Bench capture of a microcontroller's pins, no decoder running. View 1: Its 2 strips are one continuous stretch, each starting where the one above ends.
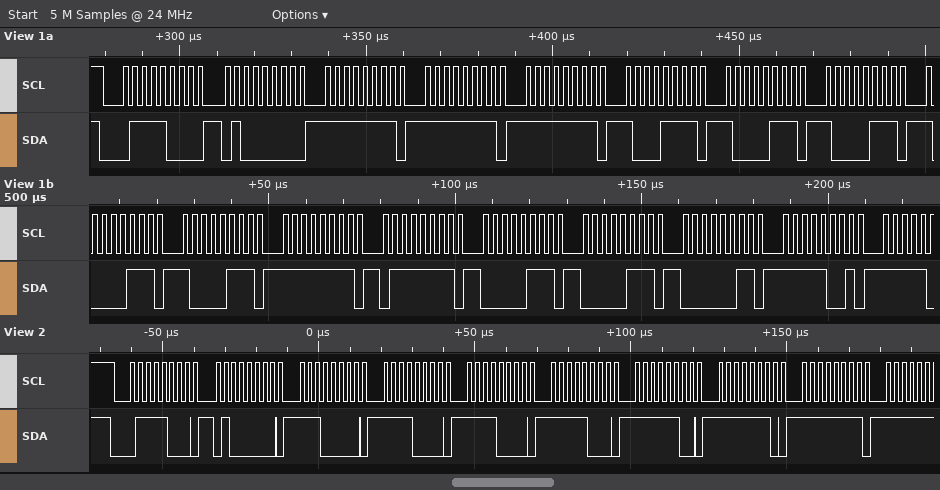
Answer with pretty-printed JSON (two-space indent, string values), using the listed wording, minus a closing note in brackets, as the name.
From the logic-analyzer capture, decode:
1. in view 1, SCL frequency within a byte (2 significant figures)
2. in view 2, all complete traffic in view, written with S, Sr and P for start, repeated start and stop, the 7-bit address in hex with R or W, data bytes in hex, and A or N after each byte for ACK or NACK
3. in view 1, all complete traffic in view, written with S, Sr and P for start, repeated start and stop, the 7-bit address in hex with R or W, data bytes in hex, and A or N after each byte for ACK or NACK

{
  "in view 1, SCL frequency within a byte": "400 kHz",
  "in view 2, all complete traffic in view, written with S, Sr and P for start, repeated start and stop, the 7-bit address in hex with R or W, data bytes in hex, and A or N after each byte for ACK or NACK": "S 3CW A 40 A E0 A F0 A F0 A F8 A FC A FE A FF A",
  "in view 1, all complete traffic in view, written with S, Sr and P for start, repeated start and stop, the 7-bit address in hex with R or W, data bytes in hex, and A or N after each byte for ACK or NACK": "S 3CW A 40 A FF A FF A FF A 8F A 87 A 87 A 87 A 87 A FF A 7F A 07 A 07 A 03 A F9 A"
}
